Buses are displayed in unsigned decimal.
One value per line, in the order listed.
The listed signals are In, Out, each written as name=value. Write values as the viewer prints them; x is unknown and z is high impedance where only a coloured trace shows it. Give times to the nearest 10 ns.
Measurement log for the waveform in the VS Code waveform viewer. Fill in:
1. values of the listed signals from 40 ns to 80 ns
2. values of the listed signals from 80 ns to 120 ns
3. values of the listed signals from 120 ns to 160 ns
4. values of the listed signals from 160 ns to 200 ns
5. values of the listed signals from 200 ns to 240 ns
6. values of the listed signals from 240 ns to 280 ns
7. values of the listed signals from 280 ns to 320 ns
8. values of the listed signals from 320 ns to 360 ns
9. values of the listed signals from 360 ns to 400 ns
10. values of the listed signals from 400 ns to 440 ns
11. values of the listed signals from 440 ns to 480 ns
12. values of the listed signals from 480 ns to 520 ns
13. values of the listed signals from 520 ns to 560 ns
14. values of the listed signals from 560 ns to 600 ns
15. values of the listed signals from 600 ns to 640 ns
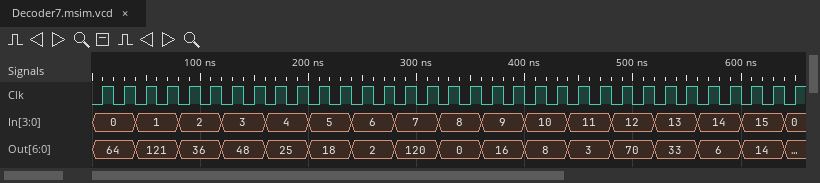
In=1, Out=121
In=2, Out=36
In=3, Out=48
In=4, Out=25
In=5, Out=18
In=6, Out=2
In=7, Out=120
In=8, Out=0
In=9, Out=16
In=10, Out=8
In=11, Out=3
In=12, Out=70
In=13, Out=33
In=14, Out=6
In=15, Out=14
